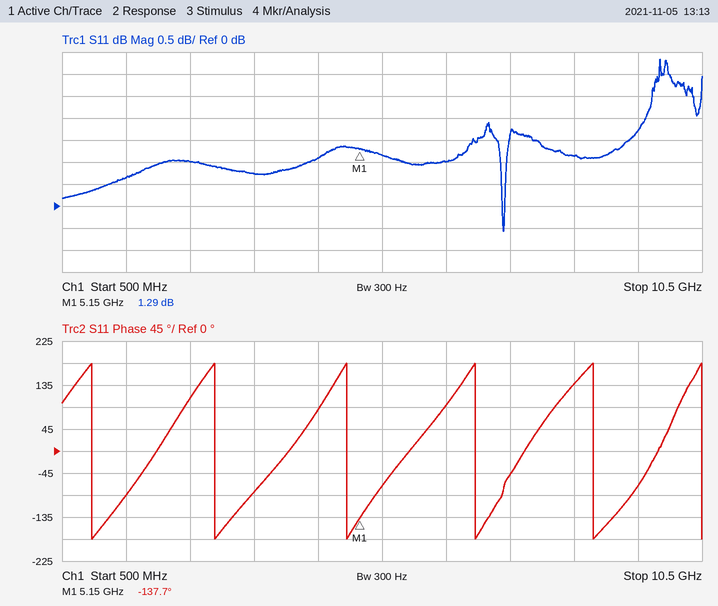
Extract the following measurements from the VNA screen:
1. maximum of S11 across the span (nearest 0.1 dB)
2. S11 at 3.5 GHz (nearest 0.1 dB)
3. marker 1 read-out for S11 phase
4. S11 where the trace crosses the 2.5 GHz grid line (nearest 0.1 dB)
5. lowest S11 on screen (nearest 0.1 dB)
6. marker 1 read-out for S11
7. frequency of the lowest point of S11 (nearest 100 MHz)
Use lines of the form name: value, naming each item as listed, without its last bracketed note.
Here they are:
maximum of S11 across the span: 3.3 dB
S11 at 3.5 GHz: 0.7 dB
marker 1 read-out for S11 phase: -137.7°
S11 where the trace crosses the 2.5 GHz grid line: 1.0 dB
lowest S11 on screen: -0.6 dB
marker 1 read-out for S11: 1.29 dB
frequency of the lowest point of S11: 7.4 GHz
